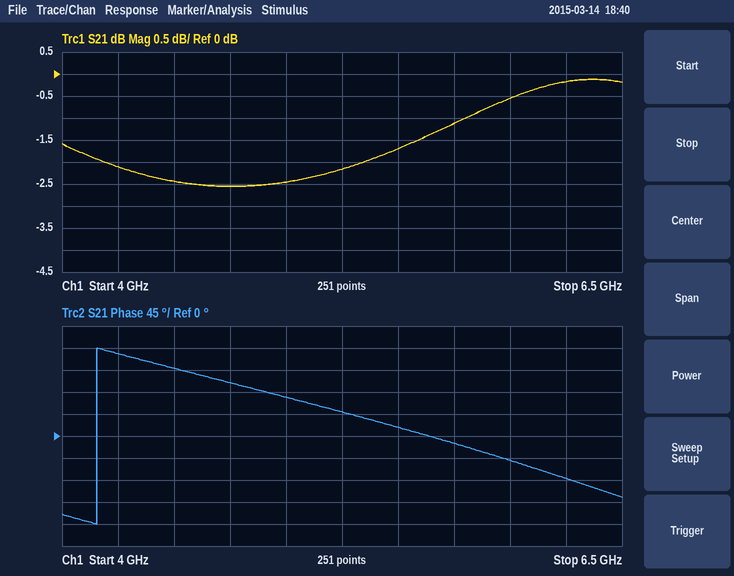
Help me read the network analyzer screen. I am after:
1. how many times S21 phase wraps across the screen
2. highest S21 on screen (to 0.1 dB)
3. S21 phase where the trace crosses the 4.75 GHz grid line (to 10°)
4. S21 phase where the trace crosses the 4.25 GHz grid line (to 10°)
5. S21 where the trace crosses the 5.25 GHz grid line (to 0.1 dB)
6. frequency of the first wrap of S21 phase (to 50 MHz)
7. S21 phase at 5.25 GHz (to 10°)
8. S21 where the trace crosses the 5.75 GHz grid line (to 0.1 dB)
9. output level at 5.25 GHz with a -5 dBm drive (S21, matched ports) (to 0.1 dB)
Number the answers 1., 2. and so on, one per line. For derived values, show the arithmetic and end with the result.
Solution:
1. 1
2. -0.1 dB
3. 110°
4. 170°
5. -2.2 dB
6. 4.15 GHz
7. 50°
8. -1.1 dB
9. -5 dBm + (-2.2 dB) = -7.2 dBm
